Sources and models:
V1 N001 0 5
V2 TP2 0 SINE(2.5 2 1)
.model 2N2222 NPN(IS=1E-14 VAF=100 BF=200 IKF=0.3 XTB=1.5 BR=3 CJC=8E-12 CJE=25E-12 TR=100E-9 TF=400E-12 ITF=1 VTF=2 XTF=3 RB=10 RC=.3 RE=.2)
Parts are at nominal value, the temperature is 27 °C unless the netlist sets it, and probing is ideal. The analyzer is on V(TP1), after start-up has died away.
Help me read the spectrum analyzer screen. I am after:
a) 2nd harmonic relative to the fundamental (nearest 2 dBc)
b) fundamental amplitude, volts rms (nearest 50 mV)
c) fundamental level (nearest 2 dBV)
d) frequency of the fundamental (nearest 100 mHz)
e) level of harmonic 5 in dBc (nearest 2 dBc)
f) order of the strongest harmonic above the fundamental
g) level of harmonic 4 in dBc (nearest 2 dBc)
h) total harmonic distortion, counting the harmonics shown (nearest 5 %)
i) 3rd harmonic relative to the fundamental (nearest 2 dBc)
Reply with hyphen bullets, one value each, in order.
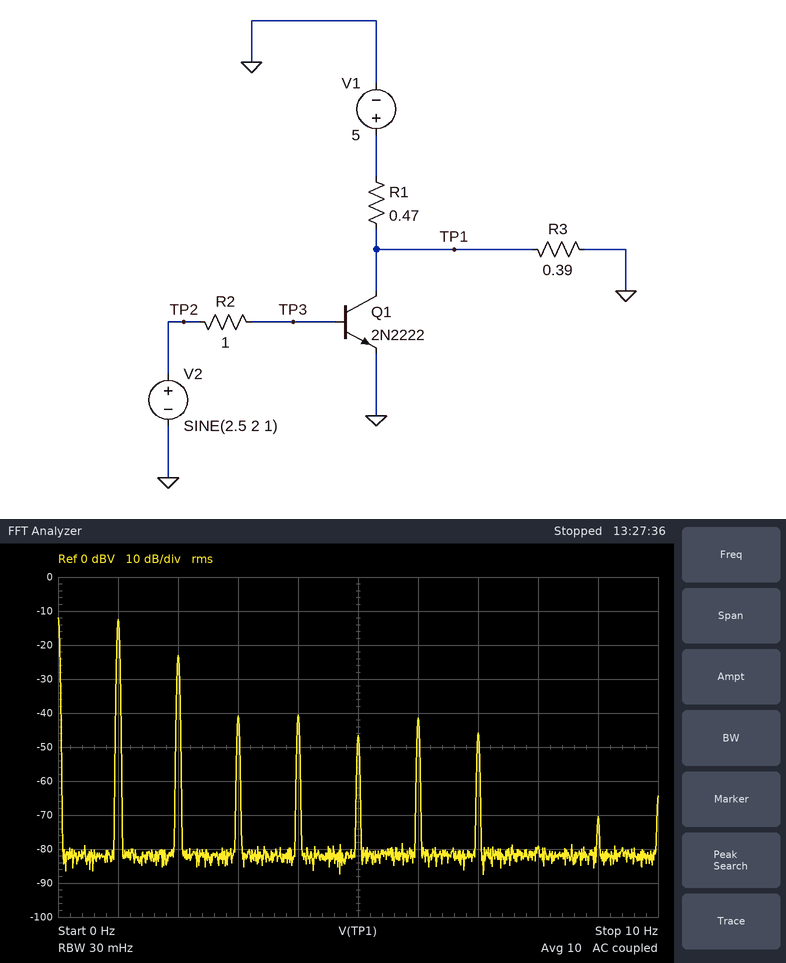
- -10 dBc
- 250 mV
- -12 dBV
- 1.0 Hz
- -34 dBc
- 2
- -28 dBc
- 30 %
- -28 dBc
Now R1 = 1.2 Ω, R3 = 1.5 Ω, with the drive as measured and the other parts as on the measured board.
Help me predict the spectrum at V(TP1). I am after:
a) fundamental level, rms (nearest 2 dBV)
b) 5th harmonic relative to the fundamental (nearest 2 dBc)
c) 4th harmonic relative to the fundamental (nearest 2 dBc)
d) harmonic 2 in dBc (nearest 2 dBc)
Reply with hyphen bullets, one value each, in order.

- -6 dBV
- -24 dBc
- -20 dBc
- -6 dBc
